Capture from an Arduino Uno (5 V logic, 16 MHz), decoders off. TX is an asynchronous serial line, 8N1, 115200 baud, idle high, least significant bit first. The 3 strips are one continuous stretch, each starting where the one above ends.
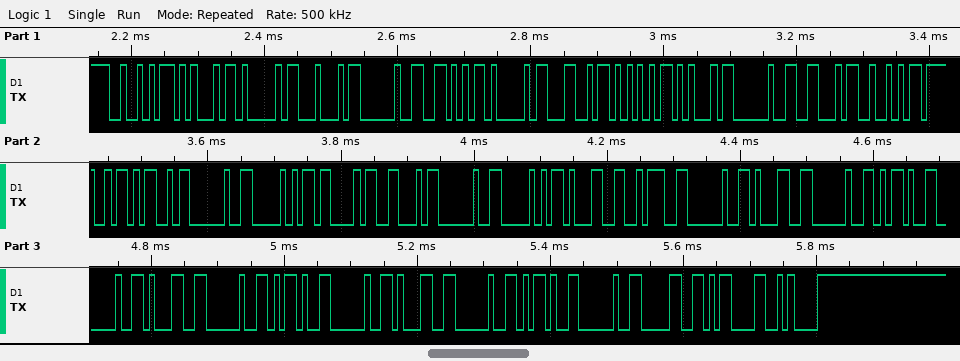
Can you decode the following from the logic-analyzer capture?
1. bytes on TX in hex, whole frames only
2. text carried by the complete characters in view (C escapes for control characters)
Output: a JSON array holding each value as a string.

["52 45 41 44 20 56 41 4C 55 45 20 46 52 4F 4D 20 50 43 46 20 50 31 3A 20 31 20 2D 20 31 20 2D 20 31 20 2D 20 30 0D 0A", "\"READ VALUE FROM PCF P1: 1 - 1 - 1 - 0\\r\\n\""]
